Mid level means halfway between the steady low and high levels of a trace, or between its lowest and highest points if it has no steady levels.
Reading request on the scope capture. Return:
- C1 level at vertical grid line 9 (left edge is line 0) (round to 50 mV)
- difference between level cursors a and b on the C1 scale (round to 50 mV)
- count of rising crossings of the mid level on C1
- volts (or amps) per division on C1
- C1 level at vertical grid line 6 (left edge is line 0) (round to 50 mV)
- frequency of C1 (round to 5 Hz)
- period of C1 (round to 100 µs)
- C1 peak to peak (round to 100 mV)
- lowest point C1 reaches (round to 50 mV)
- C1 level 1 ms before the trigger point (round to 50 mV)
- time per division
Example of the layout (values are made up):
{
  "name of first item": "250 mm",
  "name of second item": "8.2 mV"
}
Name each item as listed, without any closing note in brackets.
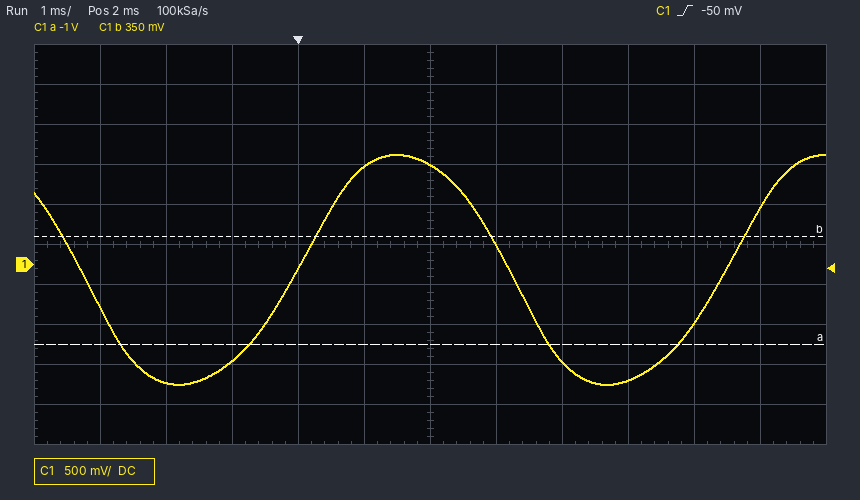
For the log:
{
  "C1 level at vertical grid line 9 (left edge is line 0)": "-1.45 V",
  "difference between level cursors a and b on the C1 scale": "1.35 V",
  "count of rising crossings of the mid level on C1": "2",
  "volts (or amps) per division on C1": "500 mV",
  "C1 level at vertical grid line 6 (left edge is line 0)": "1.25 V",
  "frequency of C1": "155 Hz",
  "period of C1": "6.5 ms",
  "C1 peak to peak": "2.90 V",
  "lowest point C1 reaches": "-1.50 V",
  "C1 level 1 ms before the trigger point": "-1.20 V",
  "time per division": "1 ms"
}
